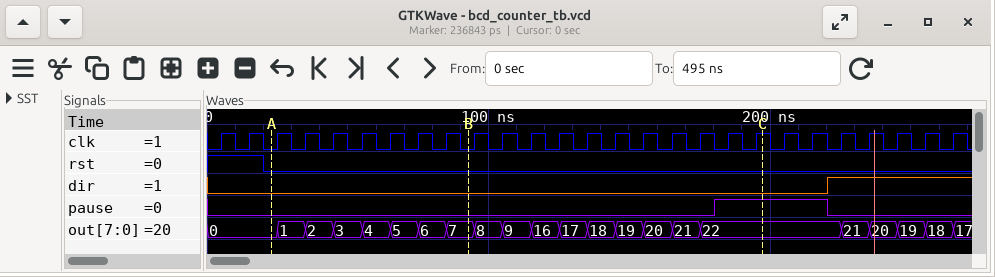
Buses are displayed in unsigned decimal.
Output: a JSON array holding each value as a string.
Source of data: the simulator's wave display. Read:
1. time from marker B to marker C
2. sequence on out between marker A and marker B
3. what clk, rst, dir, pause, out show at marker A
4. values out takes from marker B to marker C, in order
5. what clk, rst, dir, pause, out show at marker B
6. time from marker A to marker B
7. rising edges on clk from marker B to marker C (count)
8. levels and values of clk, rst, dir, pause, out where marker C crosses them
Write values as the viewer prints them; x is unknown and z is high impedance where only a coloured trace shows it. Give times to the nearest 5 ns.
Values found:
["105 ns", "0, 1, 2, 3, 4, 5, 6, 7", "clk=0, rst=0, dir=0, pause=0, out=0", "7, 8, 9, 16, 17, 18, 19, 20, 21, 22", "clk=0, rst=0, dir=0, pause=0, out=7", "70 ns", "11", "clk=1, rst=0, dir=0, pause=1, out=22"]
